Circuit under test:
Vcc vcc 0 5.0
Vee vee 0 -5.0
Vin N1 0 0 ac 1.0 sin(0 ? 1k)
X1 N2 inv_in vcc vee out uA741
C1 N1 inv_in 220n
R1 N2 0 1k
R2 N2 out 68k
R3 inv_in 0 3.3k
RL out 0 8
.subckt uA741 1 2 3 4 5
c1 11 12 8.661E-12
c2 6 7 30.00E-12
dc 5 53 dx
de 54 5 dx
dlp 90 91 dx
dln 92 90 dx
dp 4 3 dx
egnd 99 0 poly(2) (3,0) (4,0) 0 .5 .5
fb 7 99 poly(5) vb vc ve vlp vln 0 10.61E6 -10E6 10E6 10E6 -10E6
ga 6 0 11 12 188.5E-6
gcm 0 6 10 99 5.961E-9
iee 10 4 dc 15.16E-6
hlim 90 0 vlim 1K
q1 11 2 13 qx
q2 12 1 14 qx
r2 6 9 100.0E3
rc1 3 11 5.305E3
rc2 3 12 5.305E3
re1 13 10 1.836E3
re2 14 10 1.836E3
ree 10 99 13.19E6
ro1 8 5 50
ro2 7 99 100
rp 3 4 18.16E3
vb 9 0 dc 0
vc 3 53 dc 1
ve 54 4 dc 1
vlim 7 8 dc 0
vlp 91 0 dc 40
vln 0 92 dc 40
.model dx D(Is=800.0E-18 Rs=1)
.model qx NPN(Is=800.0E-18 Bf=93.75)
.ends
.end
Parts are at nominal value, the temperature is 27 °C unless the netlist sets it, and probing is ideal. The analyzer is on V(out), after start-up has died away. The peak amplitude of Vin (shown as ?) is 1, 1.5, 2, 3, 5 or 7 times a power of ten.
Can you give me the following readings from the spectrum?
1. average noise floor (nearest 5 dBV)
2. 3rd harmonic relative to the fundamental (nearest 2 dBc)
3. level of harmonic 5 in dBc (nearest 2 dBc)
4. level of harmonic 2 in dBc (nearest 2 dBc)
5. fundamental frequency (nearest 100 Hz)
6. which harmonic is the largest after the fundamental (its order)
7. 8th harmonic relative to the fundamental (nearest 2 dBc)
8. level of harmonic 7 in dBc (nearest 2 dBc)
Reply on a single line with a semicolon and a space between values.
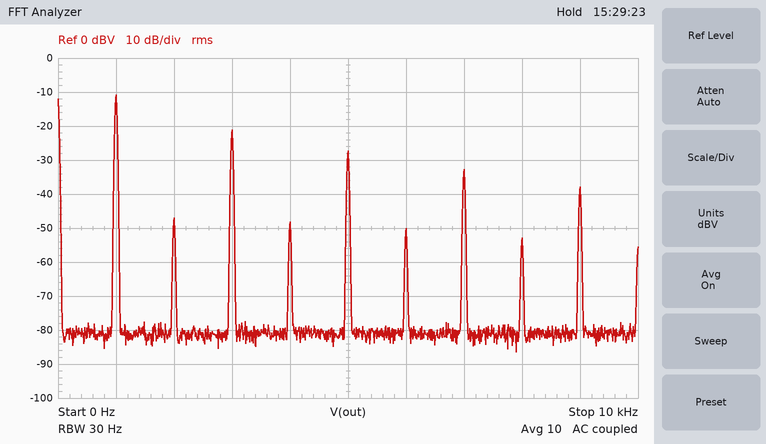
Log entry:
-80 dBV; -10 dBc; -16 dBc; -36 dBc; 1.0 kHz; 3; -42 dBc; -22 dBc
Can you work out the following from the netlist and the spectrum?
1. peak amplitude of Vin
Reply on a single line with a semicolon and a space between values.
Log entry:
15 mV
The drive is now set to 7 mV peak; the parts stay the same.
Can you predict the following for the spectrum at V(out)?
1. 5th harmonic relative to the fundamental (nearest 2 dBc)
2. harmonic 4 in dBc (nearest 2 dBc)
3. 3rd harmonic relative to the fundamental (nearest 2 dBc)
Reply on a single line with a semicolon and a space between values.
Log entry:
-20 dBc; -28 dBc; -12 dBc
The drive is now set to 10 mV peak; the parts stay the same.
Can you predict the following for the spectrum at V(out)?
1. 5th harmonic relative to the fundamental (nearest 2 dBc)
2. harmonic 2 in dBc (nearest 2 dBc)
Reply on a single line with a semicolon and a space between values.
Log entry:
-18 dBc; -32 dBc
